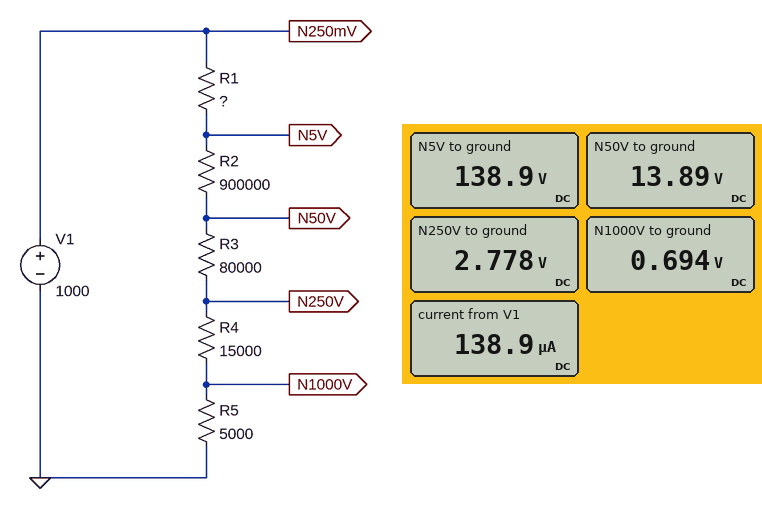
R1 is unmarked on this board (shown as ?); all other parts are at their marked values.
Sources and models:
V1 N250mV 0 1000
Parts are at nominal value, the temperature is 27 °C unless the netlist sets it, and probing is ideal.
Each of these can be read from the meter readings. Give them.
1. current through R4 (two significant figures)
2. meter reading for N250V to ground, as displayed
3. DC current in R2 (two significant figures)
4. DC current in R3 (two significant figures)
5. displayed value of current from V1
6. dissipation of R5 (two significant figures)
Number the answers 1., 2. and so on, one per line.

1. 140 µA
2. 2.778 V
3. 140 µA
4. 140 µA
5. 138.9 µA
6. 96 µW
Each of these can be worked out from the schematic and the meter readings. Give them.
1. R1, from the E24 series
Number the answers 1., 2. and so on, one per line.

1. 6.2 MΩ
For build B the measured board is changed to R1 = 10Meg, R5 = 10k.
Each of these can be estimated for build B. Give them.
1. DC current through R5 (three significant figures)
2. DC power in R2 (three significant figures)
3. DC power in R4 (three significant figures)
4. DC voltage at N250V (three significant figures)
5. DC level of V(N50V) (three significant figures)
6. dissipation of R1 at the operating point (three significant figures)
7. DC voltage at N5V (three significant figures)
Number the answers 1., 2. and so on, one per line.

1. 90.9 µA
2. 7.43 mW
3. 124 µW
4. 2.27 V
5. 9.54 V
6. 82.6 mW
7. 91.3 V
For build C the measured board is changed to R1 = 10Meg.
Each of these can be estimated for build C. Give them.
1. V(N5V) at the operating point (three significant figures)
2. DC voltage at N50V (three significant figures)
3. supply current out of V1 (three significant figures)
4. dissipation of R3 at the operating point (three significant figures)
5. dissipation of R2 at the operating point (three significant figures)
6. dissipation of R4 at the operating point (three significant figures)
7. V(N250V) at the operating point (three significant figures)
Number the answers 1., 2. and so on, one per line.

1. 90.9 V
2. 9.09 V
3. 90.9 µA
4. 661 µW
5. 7.44 mW
6. 124 µW
7. 1.82 V
